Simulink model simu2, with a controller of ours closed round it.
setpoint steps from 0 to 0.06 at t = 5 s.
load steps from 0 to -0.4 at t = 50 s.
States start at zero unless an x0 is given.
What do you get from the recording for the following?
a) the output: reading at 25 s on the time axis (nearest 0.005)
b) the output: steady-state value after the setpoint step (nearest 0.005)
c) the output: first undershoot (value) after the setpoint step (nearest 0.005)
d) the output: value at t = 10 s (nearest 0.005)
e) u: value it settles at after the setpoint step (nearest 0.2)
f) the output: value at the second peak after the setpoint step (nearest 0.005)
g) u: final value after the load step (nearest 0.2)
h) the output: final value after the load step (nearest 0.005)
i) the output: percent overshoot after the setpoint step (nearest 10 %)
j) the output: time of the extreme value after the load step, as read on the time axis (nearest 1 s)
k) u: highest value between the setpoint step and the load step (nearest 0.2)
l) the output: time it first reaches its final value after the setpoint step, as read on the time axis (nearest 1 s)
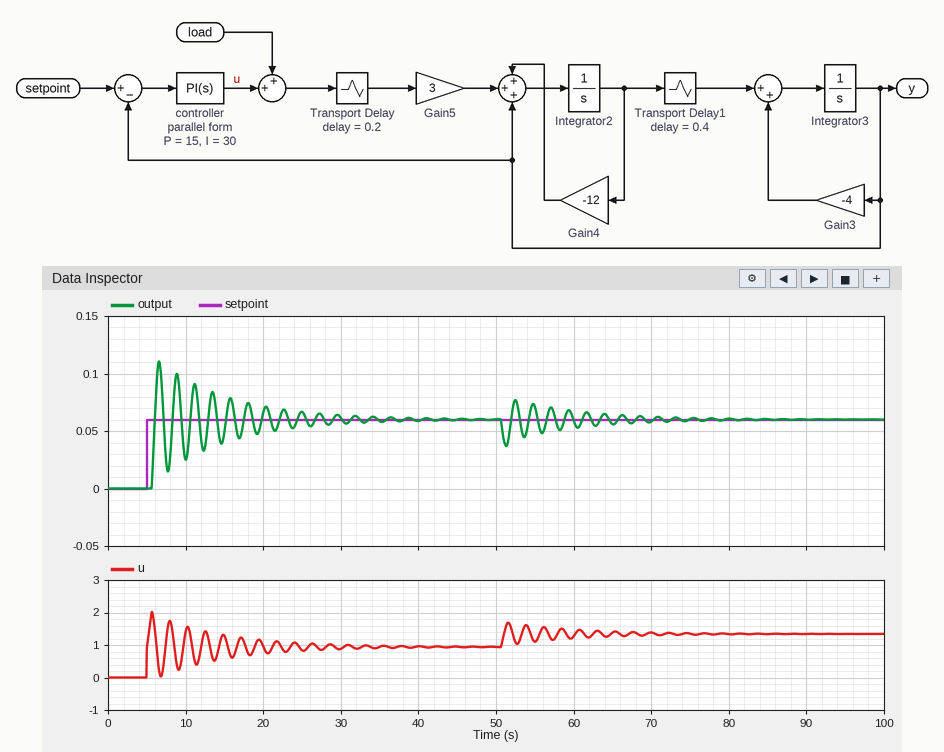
0.065
0.060
0.015
0.025
1.0
0.100
1.4
0.060
80 %
51 s
2.0
6 s
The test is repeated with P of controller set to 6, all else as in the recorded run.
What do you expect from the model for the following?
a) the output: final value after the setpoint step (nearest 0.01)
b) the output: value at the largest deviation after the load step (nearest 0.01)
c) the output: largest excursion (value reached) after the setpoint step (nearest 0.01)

0.06
0.04
0.11
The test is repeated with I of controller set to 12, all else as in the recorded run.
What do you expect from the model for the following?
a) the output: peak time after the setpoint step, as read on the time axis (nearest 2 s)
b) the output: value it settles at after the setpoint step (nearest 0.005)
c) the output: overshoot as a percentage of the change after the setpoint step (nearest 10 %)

6 s
0.060
20 %
